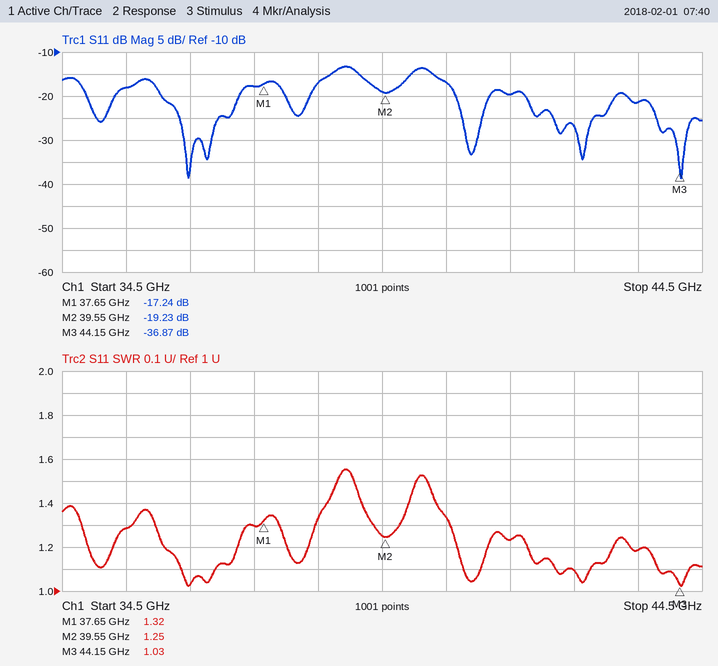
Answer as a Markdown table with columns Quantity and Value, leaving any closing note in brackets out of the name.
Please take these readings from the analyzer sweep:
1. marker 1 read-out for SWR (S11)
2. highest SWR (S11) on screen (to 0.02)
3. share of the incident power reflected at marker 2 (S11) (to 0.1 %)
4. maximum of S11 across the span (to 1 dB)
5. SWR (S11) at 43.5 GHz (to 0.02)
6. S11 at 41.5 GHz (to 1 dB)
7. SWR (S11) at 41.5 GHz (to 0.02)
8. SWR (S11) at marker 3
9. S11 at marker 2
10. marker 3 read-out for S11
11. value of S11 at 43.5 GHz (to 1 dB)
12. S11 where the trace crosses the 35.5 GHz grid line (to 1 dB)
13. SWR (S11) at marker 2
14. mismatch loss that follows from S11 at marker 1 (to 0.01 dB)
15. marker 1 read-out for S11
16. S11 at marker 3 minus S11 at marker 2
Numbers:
| Quantity | Value |
|---|---|
| marker 1 read-out for SWR | 1.32 |
| highest SWR (S11) on screen | 1.56 |
| share of the incident power reflected at marker 2 (S11) | 1.2 % |
| maximum of S11 across the span | -13 dB |
| SWR (S11) at 43.5 GHz | 1.18 |
| S11 at 41.5 GHz | -20 dB |
| SWR (S11) at 41.5 GHz | 1.24 |
| SWR (S11) at marker 3 | 1.03 |
| S11 at marker 2 | -19.23 dB |
| marker 3 read-out for S11 | -36.87 dB |
| value of S11 at 43.5 GHz | -21 dB |
| S11 where the trace crosses the 35.5 GHz grid line | -18 dB |
| SWR (S11) at marker 2 | 1.25 |
| mismatch loss that follows from S11 at marker 1 | 0.08 dB |
| marker 1 read-out for S11 | -17.24 dB |
| S11 at marker 3 minus S11 at marker 2 | -17.64 dB |
